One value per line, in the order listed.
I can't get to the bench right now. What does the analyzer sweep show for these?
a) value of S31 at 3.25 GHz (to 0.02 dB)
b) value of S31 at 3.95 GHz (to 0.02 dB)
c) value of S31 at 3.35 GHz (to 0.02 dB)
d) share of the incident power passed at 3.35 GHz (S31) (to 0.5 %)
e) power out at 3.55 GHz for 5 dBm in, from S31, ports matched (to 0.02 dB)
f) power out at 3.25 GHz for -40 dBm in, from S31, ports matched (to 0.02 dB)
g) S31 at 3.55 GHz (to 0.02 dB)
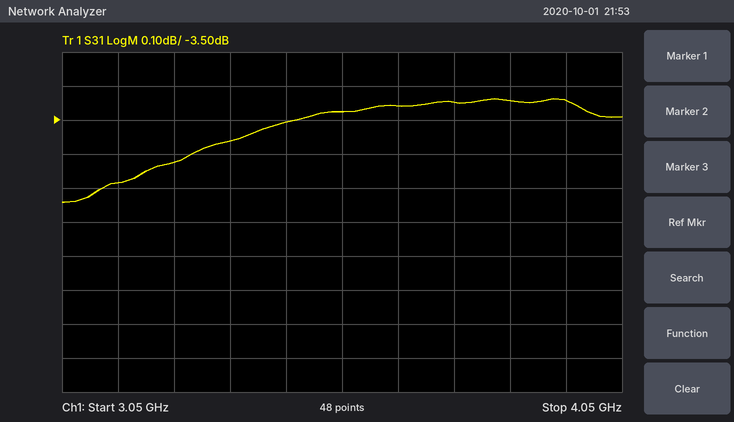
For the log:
-3.62 dB
-3.44 dB
-3.56 dB
44.0 %
1.52 dBm
-43.62 dBm
-3.48 dB
